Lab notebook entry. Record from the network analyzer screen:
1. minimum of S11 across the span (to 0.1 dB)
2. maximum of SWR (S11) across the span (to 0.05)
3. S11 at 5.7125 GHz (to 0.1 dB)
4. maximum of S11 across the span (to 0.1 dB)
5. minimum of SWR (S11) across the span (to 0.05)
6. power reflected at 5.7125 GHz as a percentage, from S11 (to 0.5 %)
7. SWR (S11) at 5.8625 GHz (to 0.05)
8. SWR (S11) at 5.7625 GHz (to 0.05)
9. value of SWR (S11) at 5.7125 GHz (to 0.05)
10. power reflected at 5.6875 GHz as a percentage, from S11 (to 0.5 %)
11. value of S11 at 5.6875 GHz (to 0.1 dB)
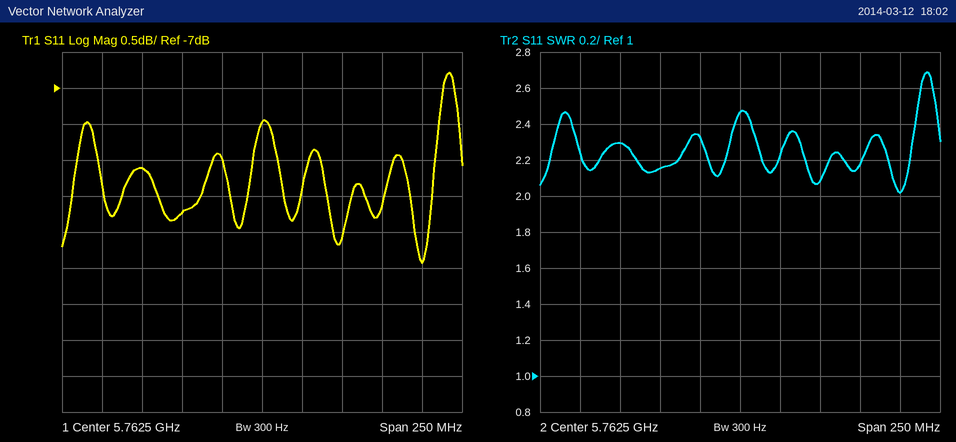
-9.4 dB
2.70
-8.7 dB
-6.8 dB
2.00
13.5 %
2.00
2.45
2.15
15.5 %
-8.1 dB
